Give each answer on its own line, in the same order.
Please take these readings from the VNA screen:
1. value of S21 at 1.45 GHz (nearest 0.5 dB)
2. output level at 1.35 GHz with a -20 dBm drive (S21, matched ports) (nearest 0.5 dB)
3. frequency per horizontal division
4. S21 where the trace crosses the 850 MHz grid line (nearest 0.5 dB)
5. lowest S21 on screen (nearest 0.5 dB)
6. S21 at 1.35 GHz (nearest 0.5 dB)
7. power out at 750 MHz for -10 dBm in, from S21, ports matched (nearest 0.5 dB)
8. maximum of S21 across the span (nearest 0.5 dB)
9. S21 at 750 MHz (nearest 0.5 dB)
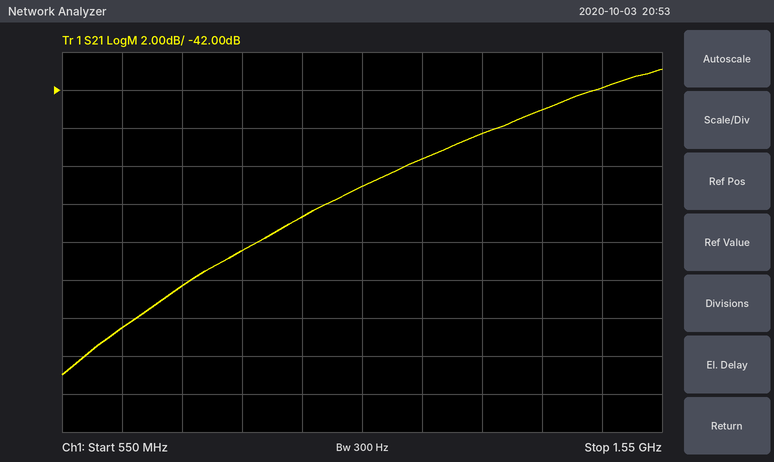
-42.0 dB
-63.0 dBm
100 MHz
-50.5 dB
-57.0 dB
-43.0 dB
-62.5 dBm
-41.0 dB
-52.5 dB
